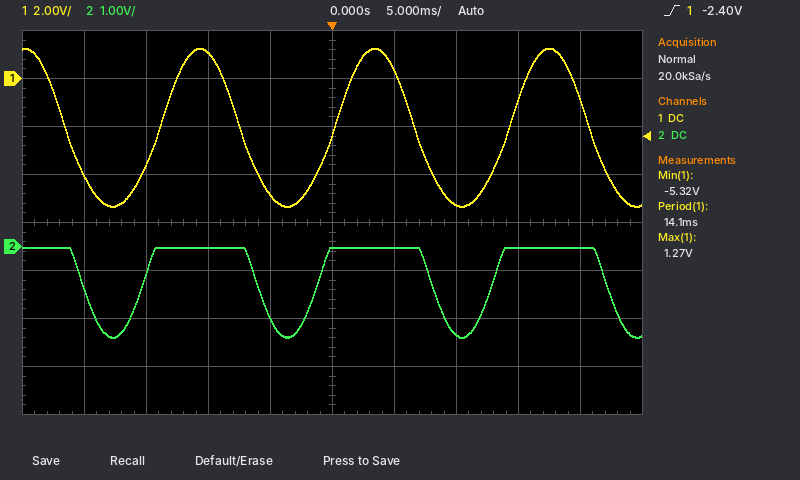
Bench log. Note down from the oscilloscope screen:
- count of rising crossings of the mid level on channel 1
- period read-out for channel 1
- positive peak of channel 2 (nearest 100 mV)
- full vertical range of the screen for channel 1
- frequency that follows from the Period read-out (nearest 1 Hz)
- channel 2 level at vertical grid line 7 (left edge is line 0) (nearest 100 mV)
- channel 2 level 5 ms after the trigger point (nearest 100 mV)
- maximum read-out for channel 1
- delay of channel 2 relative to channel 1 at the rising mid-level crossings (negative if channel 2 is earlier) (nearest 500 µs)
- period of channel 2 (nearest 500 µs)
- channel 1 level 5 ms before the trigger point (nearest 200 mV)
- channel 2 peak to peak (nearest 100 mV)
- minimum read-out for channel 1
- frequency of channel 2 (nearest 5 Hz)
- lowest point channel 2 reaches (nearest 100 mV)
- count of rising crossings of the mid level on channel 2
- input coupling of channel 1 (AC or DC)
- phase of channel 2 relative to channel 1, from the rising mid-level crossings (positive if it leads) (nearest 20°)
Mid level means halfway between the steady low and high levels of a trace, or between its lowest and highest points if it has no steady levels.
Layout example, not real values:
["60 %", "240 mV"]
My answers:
["3", "14.1 ms", "0.0 V", "16 V", "71 Hz", "-1.8 V", "0.0 V", "1.27 V", "-1.5 ms", "14.0 ms", "-4.8 V", "1.9 V", "-5.32 V", "70 Hz", "-1.9 V", "3", "DC", "+40°"]
